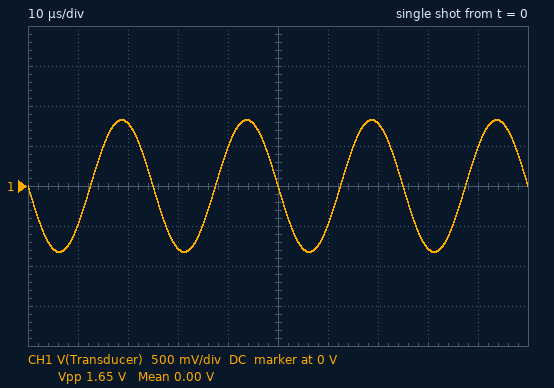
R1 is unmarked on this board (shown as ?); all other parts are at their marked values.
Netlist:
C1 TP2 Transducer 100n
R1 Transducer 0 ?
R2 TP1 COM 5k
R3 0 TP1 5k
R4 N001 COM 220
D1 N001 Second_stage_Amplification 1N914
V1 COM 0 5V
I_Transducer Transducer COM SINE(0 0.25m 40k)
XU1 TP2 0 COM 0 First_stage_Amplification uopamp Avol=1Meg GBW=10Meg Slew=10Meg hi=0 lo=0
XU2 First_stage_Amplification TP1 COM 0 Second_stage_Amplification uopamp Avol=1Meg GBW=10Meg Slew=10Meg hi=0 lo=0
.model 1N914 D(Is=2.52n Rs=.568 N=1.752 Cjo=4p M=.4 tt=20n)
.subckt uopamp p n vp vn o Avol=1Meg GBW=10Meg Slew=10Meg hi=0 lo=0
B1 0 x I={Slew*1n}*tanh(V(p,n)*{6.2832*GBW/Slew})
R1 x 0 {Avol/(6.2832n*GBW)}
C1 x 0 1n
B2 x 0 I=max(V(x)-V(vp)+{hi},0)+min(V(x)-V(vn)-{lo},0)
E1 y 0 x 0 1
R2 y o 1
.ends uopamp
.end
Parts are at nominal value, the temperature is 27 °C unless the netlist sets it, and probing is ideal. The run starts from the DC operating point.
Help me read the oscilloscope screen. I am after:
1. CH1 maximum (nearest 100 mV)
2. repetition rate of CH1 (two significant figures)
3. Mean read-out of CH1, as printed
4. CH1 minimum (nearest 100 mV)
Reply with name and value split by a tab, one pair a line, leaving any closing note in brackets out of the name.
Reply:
CH1 maximum	800 mV
repetition rate of CH1	40 kHz
Mean read-out of CH1, as printed	0.00 V
CH1 minimum	-800 mV
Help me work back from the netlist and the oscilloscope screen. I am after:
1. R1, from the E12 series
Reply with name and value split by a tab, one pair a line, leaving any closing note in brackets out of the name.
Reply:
R1, from the E12 series	3.3 kΩ
